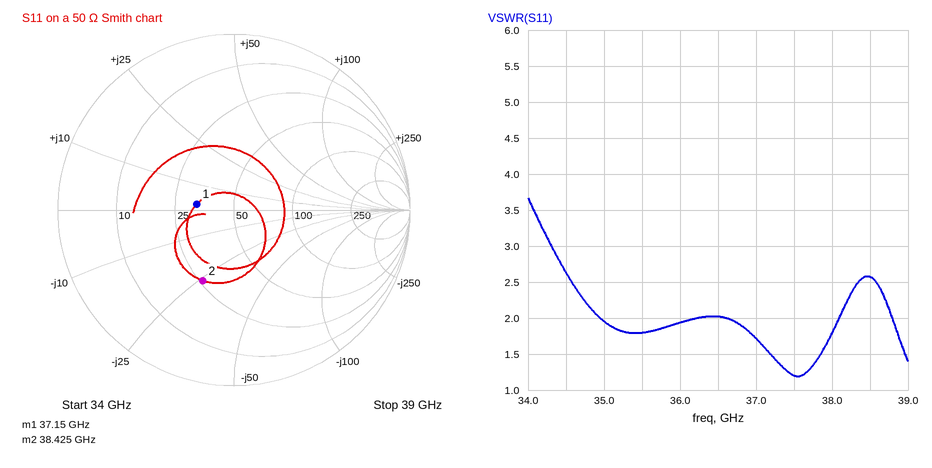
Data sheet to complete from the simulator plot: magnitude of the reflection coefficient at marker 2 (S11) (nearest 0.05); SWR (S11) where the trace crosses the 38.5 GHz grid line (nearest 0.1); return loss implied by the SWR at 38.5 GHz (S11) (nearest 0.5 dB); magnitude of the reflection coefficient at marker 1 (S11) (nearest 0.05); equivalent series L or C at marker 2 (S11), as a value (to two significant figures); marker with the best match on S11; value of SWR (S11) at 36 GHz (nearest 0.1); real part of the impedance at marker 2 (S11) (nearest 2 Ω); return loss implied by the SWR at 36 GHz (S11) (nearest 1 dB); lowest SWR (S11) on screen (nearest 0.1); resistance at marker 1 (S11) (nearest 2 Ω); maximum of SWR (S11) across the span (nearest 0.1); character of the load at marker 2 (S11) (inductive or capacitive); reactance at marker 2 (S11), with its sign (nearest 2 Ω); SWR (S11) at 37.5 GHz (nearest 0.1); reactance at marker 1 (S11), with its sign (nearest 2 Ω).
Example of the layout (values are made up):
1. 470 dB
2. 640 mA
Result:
1. 0.45
2. 2.6
3. 7.0 dB
4. 0.20
5. 160 fF
6. marker 1
7. 1.9
8. 26 Ω
9. 10 dB
10. 1.2
11. 32 Ω
12. 3.7
13. capacitive
14. -26 Ω
15. 1.2
16. +2 Ω
